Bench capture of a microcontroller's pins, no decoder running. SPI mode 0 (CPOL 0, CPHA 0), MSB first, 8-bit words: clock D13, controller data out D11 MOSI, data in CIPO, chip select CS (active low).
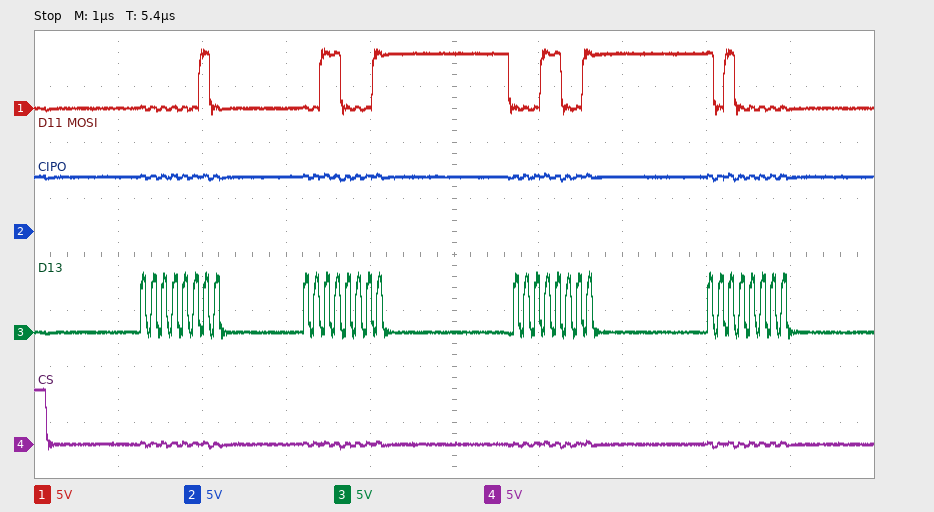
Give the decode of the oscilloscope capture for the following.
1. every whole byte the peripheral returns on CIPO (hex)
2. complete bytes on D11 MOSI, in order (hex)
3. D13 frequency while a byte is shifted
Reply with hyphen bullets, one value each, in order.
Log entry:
- FF FF FF FF
- 02 31 19 A0
- 8 MHz
